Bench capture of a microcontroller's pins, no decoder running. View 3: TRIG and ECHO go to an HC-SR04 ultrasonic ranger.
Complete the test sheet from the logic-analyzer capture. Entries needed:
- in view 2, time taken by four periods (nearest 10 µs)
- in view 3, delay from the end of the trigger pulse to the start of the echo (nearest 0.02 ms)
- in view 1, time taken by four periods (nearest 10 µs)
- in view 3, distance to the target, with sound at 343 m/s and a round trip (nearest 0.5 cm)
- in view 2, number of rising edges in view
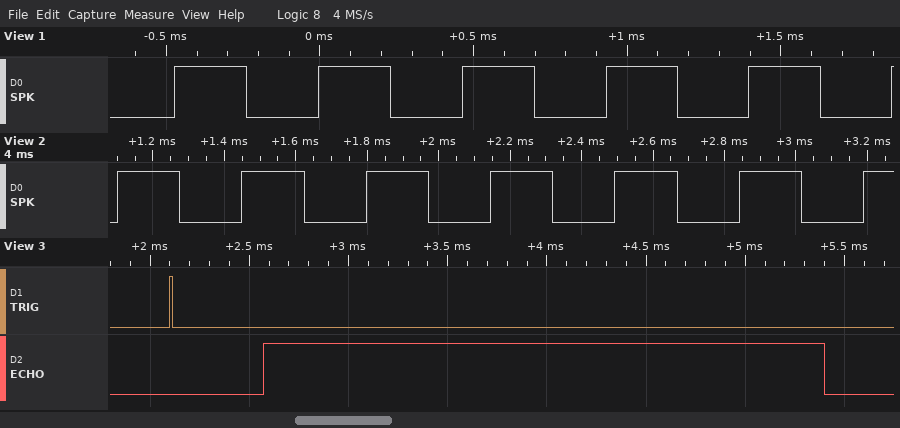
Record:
1400 µs
0.46 ms
1850 µs
48.5 cm
7
